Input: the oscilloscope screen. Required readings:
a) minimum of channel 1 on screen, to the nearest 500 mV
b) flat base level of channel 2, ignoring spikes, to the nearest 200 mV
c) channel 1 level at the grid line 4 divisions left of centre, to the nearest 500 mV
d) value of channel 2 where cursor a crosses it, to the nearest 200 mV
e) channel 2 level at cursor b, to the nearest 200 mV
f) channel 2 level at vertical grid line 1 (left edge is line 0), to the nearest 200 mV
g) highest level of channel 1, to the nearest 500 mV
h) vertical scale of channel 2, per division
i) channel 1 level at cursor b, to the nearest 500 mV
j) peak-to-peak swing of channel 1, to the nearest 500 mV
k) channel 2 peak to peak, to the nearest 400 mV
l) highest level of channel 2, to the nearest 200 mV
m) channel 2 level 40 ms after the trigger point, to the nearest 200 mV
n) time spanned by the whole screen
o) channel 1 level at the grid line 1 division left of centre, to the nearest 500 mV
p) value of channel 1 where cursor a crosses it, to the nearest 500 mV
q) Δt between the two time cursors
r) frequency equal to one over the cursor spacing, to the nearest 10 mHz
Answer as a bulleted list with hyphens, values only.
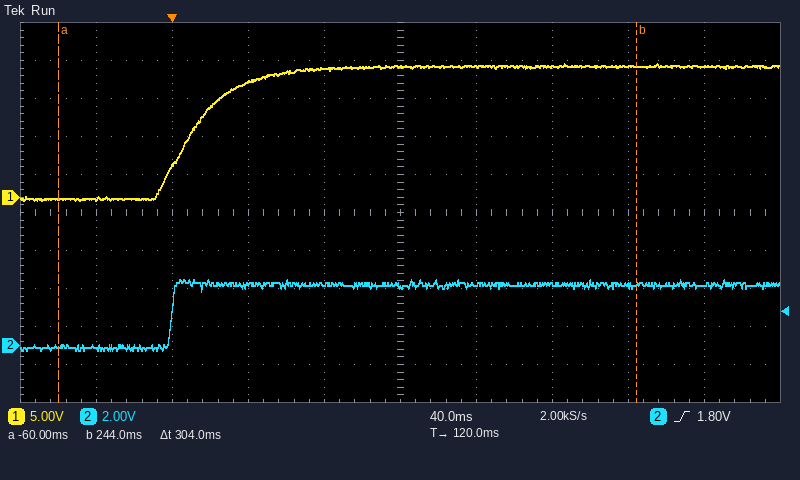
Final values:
- -500 mV
- -200 mV
- 0.0 V
- 0.0 V
- 3.2 V
- -200 mV
- 17.5 V
- 2 V
- 17.5 V
- 18.0 V
- 3.6 V
- 3.4 V
- 3.2 V
- 400 ms
- 17.0 V
- 0.0 V
- 304 ms
- 3.29 Hz
